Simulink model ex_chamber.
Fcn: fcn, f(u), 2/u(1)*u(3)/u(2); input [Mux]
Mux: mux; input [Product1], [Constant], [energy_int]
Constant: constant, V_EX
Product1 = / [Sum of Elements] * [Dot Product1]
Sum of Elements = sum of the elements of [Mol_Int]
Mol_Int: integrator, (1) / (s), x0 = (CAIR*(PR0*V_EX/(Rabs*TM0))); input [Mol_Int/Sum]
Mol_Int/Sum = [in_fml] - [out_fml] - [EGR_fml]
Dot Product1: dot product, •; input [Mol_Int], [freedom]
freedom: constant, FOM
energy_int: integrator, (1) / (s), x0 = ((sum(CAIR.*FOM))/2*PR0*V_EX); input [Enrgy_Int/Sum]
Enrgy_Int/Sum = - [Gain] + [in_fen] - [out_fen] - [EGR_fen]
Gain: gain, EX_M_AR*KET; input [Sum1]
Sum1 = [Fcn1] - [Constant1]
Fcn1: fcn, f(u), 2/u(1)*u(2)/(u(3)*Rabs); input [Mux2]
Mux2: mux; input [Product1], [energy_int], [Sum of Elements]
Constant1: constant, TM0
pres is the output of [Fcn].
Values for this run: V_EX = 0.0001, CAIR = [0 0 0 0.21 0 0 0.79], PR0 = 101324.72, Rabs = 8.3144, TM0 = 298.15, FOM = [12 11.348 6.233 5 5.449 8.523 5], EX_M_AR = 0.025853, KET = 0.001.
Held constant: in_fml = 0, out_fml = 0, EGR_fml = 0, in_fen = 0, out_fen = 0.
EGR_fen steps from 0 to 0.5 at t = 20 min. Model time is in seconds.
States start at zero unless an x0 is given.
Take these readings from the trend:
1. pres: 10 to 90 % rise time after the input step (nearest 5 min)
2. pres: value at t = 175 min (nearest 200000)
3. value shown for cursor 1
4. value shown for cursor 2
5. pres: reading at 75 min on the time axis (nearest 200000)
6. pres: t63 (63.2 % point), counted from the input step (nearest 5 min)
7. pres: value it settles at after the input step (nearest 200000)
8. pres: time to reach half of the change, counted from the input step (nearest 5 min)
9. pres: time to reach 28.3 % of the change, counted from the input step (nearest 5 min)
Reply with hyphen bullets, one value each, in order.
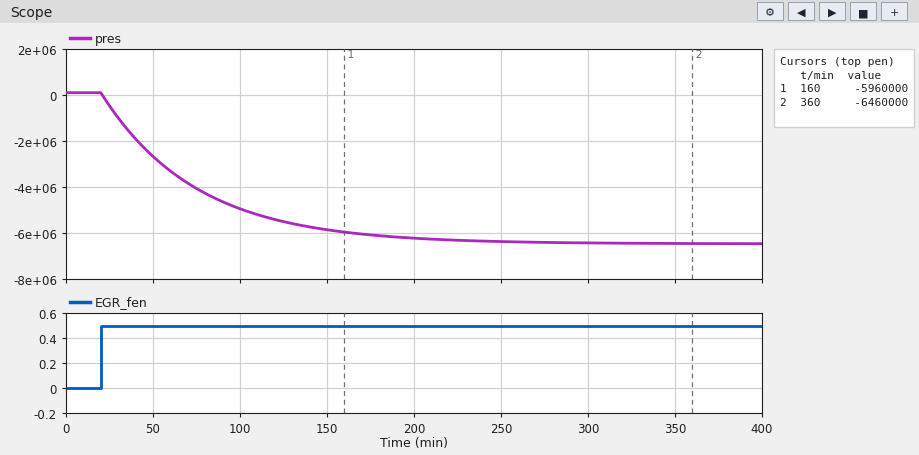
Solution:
- 120 min
- -6000000
- -5960000
- -6460000
- -4000000
- 55 min
- -6400000
- 40 min
- 20 min
